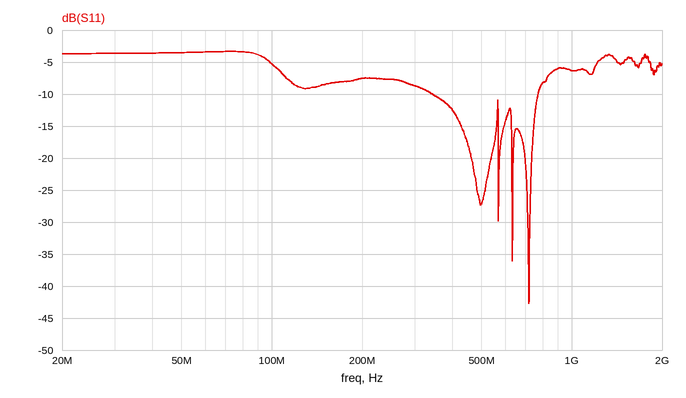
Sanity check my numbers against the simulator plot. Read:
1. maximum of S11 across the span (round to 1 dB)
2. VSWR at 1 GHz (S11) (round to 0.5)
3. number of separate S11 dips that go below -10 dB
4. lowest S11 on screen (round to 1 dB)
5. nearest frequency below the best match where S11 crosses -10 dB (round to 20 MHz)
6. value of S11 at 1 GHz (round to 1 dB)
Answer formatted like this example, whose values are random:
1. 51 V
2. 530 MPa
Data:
1. -3 dB
2. 3.0
3. 4
4. -43 dB
5. 340 MHz
6. -6 dB
